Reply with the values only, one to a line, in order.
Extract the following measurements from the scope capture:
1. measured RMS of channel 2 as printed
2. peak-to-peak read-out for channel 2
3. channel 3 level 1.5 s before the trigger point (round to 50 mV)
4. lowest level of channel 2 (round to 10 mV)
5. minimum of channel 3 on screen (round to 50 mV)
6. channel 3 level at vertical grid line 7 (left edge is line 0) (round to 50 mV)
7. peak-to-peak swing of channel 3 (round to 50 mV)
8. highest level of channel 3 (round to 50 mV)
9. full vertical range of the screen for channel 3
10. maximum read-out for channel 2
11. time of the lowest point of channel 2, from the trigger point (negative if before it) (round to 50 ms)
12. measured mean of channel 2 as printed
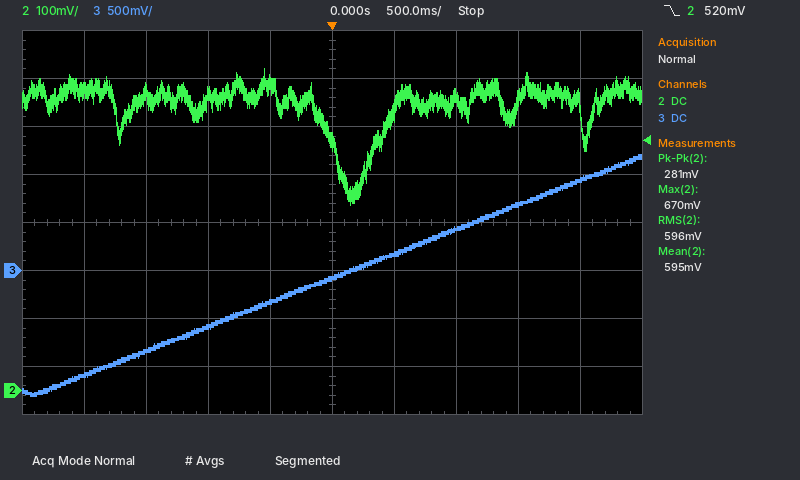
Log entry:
596 mV
281 mV
-850 mV
390 mV
-1.30 V
450 mV
2.50 V
1.20 V
4 V
670 mV
+150 ms
595 mV
